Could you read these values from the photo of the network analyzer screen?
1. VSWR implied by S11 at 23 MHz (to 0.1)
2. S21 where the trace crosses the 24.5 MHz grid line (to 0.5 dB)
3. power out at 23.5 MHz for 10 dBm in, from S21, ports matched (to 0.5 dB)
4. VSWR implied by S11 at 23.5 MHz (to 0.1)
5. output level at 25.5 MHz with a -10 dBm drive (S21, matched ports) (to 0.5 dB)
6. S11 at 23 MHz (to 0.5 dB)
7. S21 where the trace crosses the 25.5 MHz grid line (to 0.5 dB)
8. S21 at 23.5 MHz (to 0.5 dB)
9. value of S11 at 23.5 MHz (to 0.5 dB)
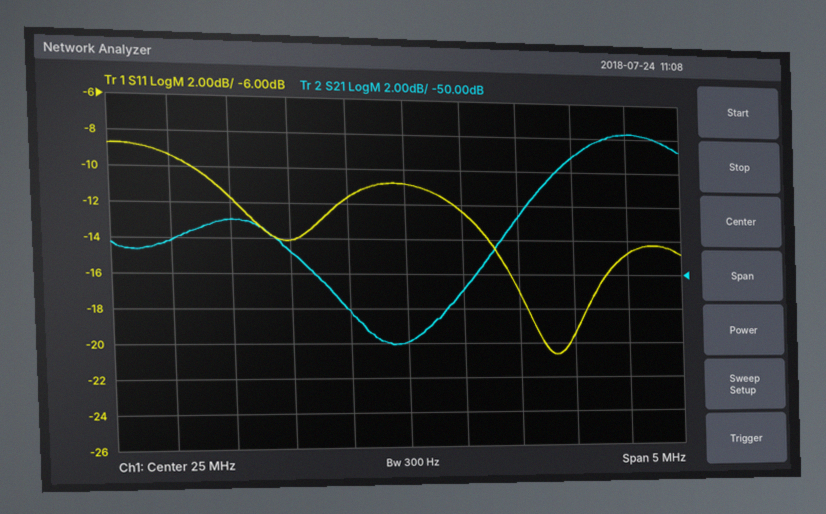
2.0
-52.0 dB
-37.0 dBm
1.7
-61.0 dBm
-9.5 dB
-51.0 dB
-47.0 dB
-11.5 dB
